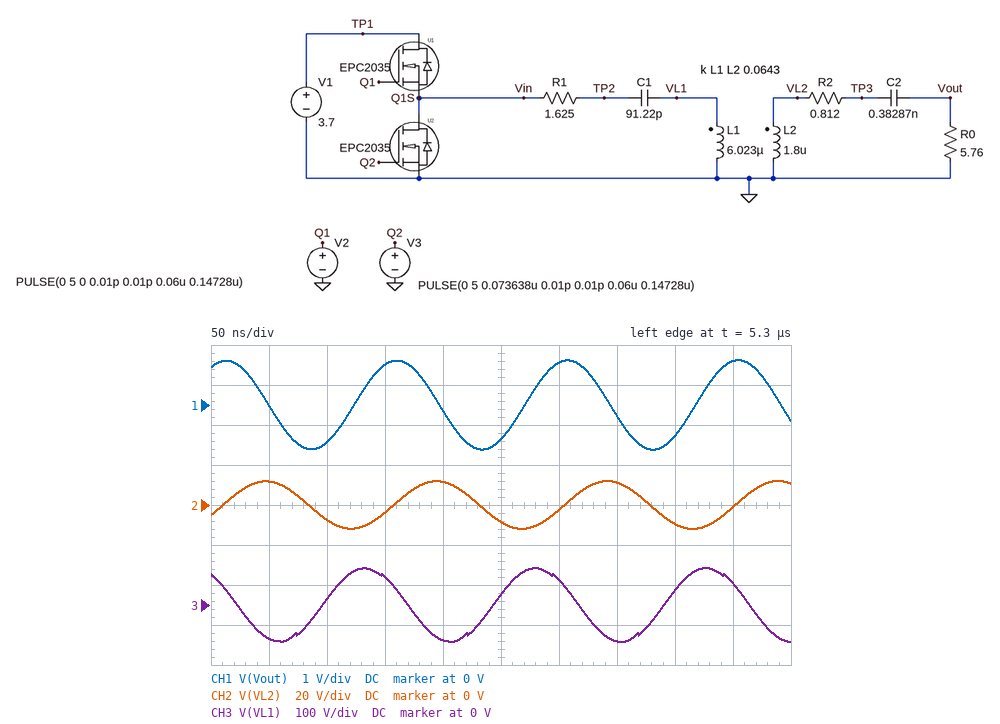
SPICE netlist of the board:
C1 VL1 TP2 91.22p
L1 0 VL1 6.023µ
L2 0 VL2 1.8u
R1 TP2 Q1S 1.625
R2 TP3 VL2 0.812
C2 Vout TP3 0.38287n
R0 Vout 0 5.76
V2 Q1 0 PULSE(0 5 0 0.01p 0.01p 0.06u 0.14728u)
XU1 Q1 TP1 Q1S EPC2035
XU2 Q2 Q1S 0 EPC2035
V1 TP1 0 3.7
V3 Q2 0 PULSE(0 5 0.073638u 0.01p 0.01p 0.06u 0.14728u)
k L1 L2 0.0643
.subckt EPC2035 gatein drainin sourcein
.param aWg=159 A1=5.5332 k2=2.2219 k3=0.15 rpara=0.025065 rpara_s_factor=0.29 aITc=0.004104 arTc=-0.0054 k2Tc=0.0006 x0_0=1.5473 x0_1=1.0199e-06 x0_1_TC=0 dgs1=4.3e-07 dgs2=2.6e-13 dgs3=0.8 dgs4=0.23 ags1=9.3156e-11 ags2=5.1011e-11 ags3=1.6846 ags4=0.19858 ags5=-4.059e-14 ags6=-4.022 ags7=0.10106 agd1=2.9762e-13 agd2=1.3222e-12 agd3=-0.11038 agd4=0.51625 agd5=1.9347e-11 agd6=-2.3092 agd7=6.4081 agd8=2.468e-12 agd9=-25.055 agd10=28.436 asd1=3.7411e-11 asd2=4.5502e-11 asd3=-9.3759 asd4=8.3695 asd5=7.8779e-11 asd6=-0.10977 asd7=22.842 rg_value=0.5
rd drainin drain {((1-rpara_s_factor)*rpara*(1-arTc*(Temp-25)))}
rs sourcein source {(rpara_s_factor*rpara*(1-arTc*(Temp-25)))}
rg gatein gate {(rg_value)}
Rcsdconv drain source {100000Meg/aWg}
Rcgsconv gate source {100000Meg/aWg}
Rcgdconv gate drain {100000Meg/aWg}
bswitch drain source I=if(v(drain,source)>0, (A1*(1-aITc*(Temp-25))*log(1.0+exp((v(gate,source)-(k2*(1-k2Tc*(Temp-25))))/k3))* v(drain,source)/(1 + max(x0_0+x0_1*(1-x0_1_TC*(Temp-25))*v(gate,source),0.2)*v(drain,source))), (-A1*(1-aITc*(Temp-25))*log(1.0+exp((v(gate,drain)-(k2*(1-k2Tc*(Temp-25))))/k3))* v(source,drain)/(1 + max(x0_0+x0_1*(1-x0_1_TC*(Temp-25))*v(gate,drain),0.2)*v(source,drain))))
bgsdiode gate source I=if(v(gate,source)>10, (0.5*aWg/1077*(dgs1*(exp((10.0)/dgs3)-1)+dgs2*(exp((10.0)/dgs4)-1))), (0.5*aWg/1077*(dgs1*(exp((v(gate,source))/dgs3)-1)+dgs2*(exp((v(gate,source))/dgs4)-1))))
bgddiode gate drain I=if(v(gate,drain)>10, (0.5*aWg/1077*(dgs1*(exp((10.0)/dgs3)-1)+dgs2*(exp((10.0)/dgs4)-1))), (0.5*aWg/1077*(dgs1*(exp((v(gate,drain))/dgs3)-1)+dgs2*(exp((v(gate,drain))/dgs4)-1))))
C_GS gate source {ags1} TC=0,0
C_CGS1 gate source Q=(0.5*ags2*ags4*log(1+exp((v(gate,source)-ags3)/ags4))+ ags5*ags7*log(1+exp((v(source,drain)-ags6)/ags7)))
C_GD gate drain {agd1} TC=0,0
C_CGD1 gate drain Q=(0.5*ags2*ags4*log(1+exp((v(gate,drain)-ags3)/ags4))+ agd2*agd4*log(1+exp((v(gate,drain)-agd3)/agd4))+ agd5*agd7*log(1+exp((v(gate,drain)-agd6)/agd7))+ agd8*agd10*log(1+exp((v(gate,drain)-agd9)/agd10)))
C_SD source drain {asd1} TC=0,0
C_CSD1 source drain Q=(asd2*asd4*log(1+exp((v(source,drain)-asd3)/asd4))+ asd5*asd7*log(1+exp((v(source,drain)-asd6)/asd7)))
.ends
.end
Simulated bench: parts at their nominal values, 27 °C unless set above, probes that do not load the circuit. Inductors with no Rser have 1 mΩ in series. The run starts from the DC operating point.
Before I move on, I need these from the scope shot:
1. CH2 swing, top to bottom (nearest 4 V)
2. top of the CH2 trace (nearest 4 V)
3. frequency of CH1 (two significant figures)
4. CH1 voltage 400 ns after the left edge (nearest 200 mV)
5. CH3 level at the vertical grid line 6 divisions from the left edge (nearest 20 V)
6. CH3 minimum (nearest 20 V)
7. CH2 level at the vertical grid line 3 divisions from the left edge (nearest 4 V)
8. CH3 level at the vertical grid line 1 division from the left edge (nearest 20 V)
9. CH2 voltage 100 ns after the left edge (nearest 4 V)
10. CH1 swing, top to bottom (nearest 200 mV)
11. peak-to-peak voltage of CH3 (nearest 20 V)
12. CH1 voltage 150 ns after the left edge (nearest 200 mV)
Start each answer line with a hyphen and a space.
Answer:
- 24 V
- 12 V
- 6.8 MHz
- -800 mV
- 60 V
- -100 V
- -4 V
- -80 V
- -8 V
- 2.2 V
- 180 V
- 1.0 V
